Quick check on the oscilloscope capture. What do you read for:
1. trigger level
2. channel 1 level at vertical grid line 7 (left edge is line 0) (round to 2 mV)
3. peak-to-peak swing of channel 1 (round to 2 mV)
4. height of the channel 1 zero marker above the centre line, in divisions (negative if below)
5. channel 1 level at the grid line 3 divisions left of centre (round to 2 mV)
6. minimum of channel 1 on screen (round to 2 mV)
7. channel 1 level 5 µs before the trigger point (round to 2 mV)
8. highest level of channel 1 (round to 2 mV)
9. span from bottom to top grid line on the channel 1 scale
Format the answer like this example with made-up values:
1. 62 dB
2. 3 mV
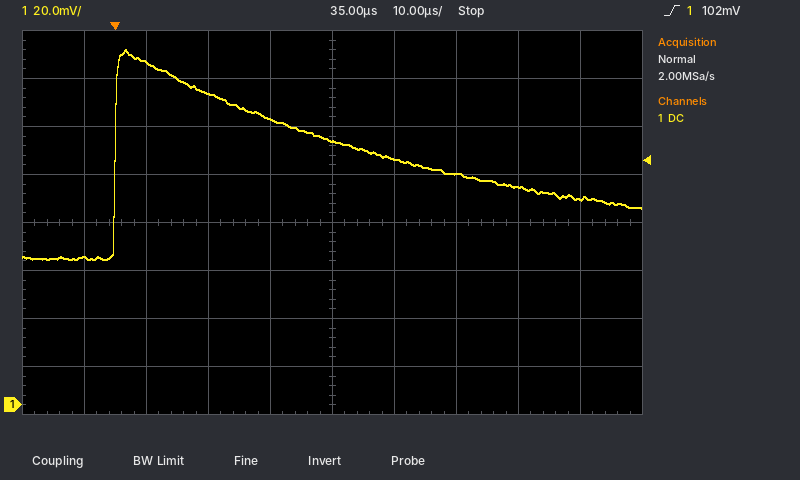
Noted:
1. 102 mV
2. 96 mV
3. 88 mV
4. -3.8 div
5. 142 mV
6. 60 mV
7. 62 mV
8. 148 mV
9. 160 mV
